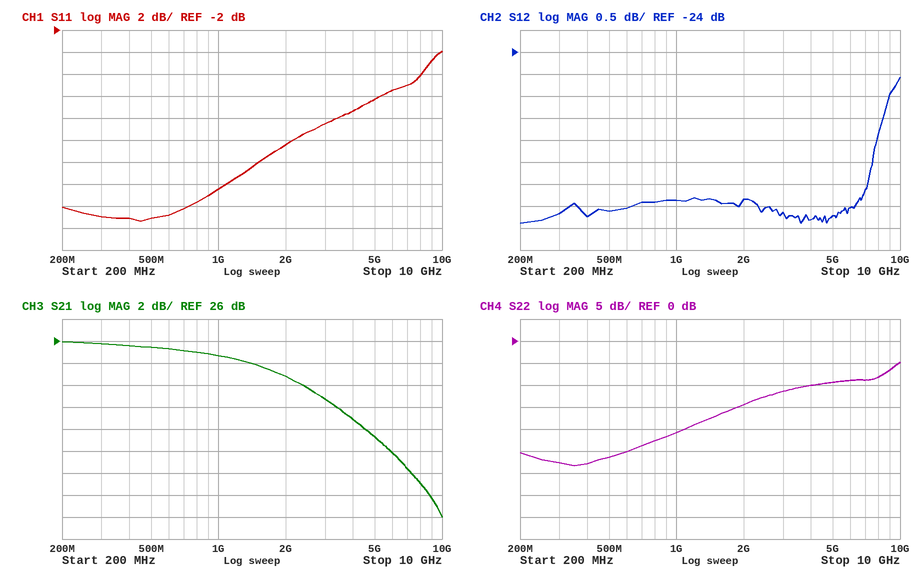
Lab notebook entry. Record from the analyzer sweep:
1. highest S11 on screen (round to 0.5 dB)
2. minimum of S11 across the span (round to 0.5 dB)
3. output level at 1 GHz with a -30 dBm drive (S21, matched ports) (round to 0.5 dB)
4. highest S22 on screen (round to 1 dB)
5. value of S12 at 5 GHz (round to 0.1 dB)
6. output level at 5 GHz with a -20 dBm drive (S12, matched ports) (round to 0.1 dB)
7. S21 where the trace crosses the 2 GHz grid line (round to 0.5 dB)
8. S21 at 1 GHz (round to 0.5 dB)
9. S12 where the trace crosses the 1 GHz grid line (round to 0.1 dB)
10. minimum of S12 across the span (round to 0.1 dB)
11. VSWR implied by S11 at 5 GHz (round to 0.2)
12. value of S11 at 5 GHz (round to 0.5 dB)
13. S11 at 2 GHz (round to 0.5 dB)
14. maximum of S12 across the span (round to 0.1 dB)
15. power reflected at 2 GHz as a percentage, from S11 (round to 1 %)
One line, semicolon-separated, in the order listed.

-4.0 dB; -19.5 dB; -5.5 dBm; -5 dB; -27.7 dB; -47.7 dBm; 23.0 dB; 24.5 dB; -27.4 dB; -27.9 dB; 2.2; -8.5 dB; -12.5 dB; -24.6 dB; 6 %
